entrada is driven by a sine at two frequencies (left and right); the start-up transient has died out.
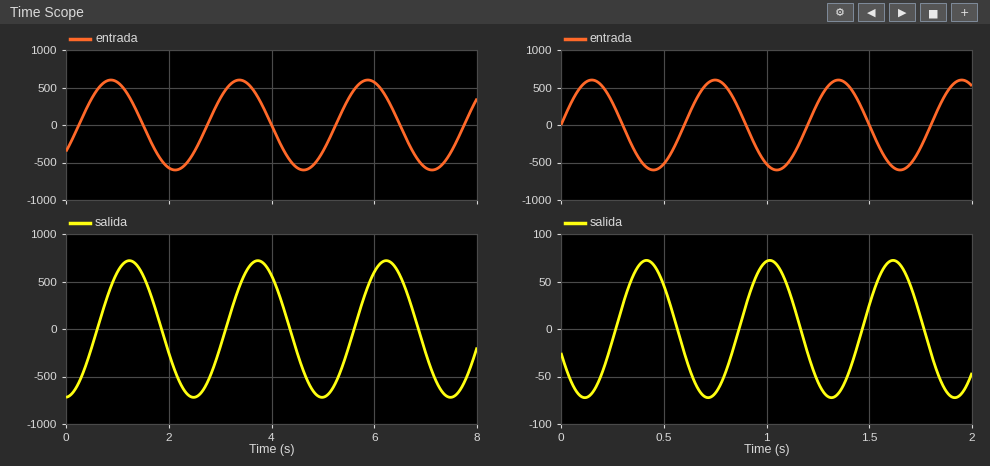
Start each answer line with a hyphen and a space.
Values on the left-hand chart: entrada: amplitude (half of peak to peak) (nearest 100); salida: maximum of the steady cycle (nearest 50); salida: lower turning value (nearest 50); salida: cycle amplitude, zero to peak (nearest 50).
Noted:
- 600
- 700
- -700
- 700
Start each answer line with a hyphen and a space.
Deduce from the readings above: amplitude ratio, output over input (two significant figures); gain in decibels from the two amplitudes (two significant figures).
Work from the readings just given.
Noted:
- 1.2
- 1.3 dB
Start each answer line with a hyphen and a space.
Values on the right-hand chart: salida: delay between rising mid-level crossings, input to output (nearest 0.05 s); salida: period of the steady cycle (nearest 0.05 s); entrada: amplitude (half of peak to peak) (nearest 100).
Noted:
- 0.25 s
- 0.60 s
- 600
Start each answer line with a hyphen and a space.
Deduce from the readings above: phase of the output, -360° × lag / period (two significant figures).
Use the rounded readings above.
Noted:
- -150°
